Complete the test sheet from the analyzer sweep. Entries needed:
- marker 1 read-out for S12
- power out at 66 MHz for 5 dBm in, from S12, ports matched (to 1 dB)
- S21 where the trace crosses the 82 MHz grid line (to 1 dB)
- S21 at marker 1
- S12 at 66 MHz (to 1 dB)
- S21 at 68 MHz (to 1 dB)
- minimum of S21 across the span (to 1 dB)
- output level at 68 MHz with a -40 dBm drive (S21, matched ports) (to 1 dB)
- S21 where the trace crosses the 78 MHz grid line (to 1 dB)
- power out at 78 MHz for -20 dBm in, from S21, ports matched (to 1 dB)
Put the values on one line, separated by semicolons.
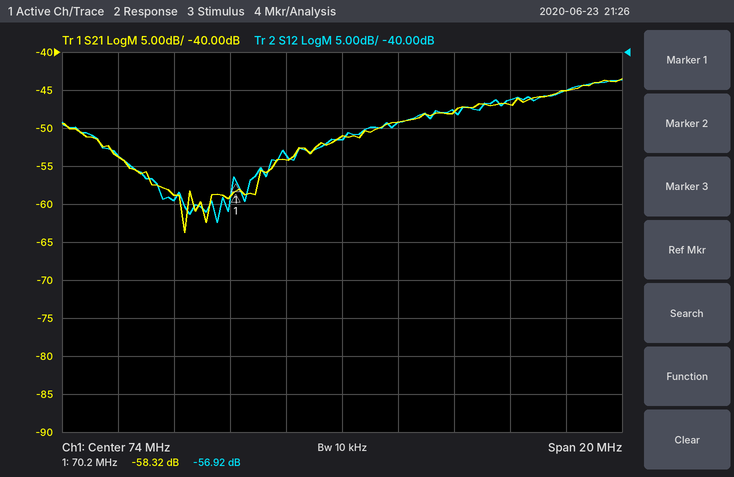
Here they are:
-56.92 dB; -49 dBm; -45 dB; -58.32 dB; -54 dB; -59 dB; -64 dB; -99 dBm; -48 dB; -68 dBm
